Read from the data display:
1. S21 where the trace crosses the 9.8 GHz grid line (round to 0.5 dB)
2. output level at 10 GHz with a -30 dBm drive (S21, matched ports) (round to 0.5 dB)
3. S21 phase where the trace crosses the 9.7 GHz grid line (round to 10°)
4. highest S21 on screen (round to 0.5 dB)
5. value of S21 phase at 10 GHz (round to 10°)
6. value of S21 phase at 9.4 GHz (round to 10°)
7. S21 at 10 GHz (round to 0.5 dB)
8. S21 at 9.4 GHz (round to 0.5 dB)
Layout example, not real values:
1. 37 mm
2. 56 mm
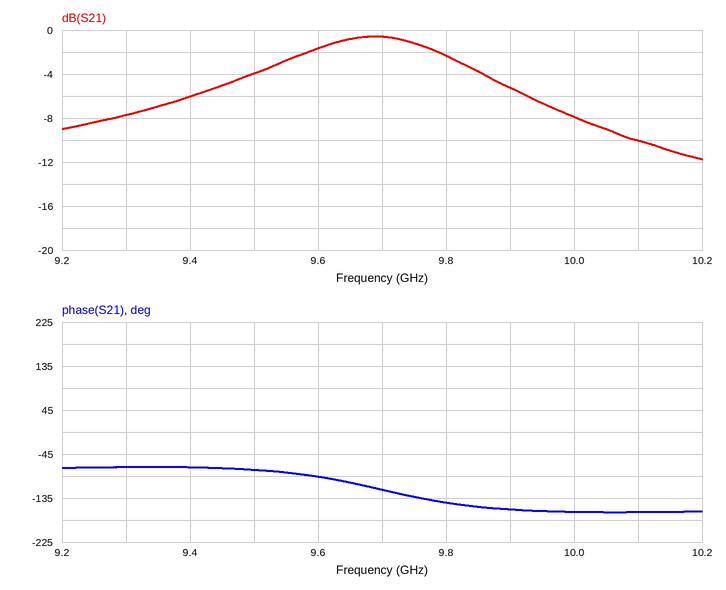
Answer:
1. -2.5 dB
2. -38.0 dBm
3. -120°
4. -0.5 dB
5. -160°
6. -70°
7. -8.0 dB
8. -6.0 dB
